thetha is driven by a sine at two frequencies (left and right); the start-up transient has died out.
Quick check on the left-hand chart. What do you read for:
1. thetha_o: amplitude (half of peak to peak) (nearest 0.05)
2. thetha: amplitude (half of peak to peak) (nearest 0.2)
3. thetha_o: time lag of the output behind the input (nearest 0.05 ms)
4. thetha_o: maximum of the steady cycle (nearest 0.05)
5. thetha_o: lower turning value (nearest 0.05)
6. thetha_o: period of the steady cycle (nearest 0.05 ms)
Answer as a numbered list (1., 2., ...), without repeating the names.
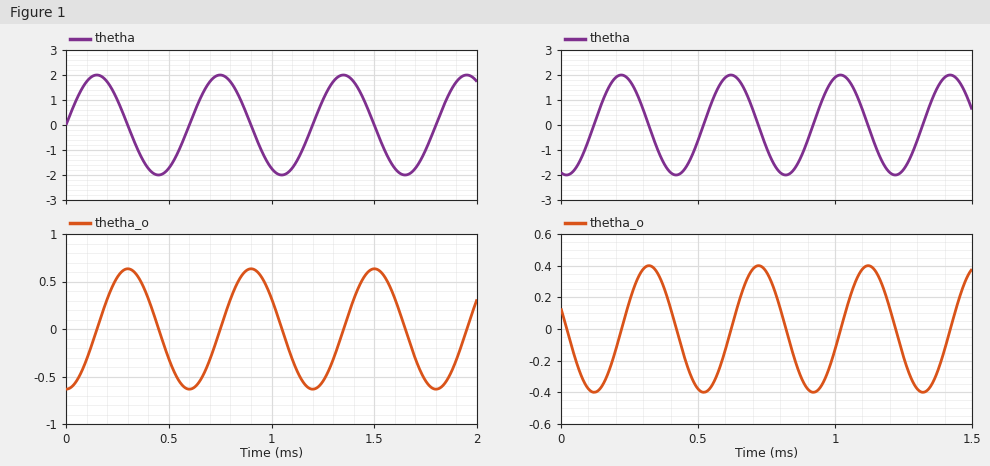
1. 0.65
2. 2.0
3. 0.15 ms
4. 0.65
5. -0.65
6. 0.60 ms
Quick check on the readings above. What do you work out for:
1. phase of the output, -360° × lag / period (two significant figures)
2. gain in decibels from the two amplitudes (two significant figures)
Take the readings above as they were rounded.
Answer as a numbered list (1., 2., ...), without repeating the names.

1. -90°
2. -9.8 dB
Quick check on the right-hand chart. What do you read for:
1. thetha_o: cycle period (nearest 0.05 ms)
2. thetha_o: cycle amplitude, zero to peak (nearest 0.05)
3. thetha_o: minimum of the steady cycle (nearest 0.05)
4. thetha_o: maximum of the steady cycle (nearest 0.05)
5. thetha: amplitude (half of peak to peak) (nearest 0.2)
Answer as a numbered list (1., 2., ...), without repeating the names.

1. 0.40 ms
2. 0.40
3. -0.40
4. 0.40
5. 2.0
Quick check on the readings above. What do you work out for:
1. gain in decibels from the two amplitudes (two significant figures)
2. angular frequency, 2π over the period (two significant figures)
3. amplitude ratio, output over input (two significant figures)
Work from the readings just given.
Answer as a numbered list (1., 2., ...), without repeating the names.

1. -14 dB
2. 16 rad/ms
3. 0.20
